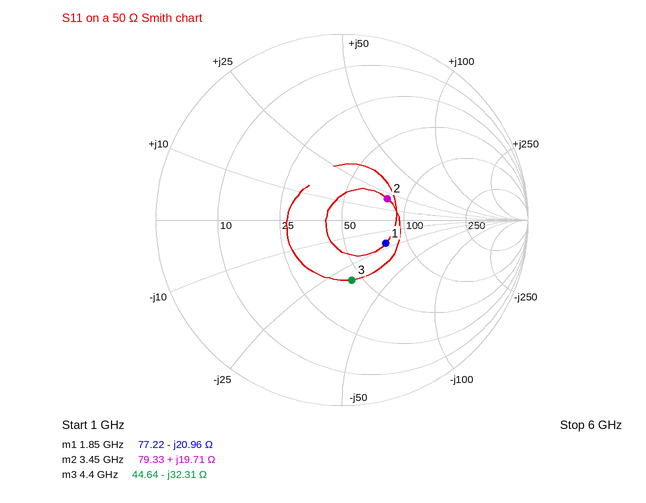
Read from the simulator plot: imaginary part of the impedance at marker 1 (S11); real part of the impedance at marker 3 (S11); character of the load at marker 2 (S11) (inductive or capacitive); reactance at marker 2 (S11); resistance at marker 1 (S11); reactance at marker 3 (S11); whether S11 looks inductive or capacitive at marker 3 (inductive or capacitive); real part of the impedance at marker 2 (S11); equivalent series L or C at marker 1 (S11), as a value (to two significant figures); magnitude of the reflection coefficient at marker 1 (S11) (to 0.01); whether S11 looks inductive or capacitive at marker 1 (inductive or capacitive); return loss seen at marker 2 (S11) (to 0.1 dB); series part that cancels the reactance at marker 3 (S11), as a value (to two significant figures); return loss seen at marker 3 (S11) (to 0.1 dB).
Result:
-20.96 Ω
44.64 Ω
inductive
+19.71 Ω
77.22 Ω
-32.31 Ω
capacitive
79.33 Ω
4.1 pF
0.27
capacitive
11.4 dB
1.2 nH
9.7 dB
